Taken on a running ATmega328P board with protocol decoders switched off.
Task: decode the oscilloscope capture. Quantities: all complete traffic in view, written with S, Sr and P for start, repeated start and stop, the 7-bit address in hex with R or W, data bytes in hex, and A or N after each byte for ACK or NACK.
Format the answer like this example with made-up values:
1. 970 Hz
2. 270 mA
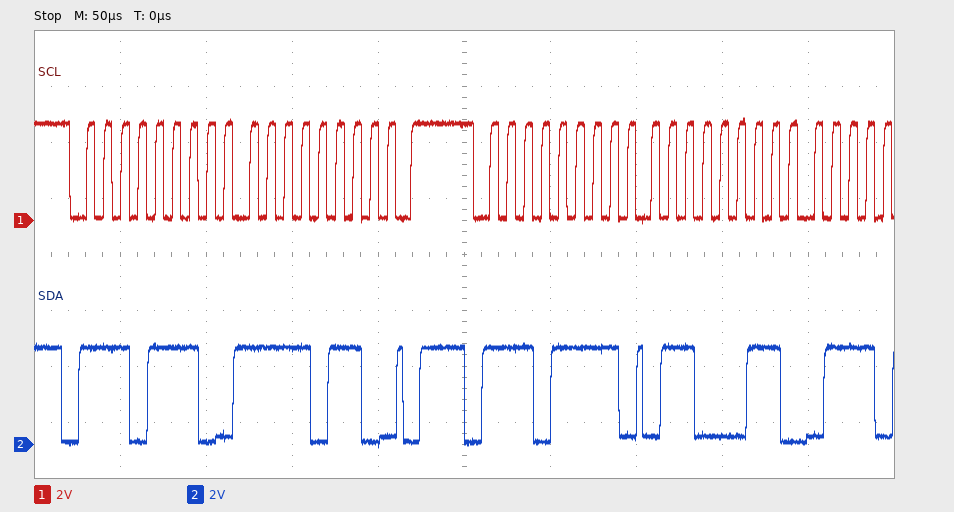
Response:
1. S 77W A F6 A P S 77R A 63 A
